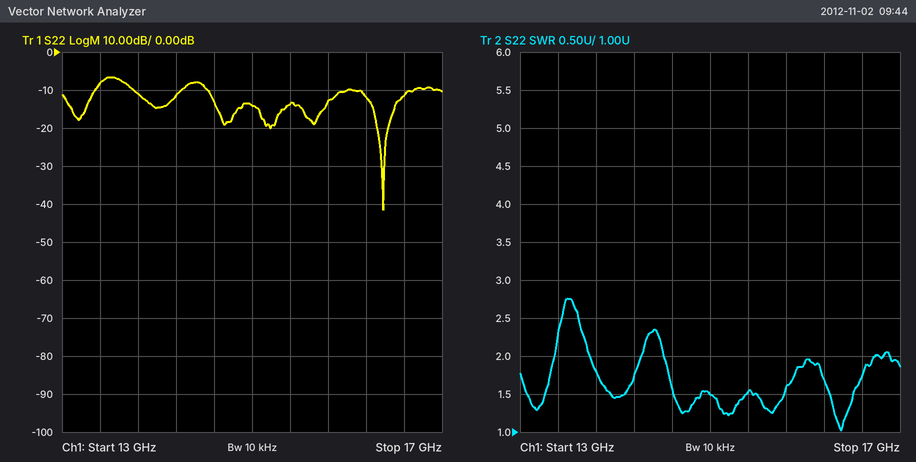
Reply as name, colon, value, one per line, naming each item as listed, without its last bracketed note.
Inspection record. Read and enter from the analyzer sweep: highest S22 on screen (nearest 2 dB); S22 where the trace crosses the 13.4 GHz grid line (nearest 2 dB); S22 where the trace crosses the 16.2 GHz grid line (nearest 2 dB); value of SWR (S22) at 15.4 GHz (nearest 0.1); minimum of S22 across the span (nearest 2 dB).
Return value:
highest S22 on screen: -6 dB
S22 where the trace crosses the 13.4 GHz grid line: -8 dB
S22 where the trace crosses the 16.2 GHz grid line: -12 dB
value of SWR (S22) at 15.4 GHz: 1.5
minimum of S22 across the span: -42 dB
